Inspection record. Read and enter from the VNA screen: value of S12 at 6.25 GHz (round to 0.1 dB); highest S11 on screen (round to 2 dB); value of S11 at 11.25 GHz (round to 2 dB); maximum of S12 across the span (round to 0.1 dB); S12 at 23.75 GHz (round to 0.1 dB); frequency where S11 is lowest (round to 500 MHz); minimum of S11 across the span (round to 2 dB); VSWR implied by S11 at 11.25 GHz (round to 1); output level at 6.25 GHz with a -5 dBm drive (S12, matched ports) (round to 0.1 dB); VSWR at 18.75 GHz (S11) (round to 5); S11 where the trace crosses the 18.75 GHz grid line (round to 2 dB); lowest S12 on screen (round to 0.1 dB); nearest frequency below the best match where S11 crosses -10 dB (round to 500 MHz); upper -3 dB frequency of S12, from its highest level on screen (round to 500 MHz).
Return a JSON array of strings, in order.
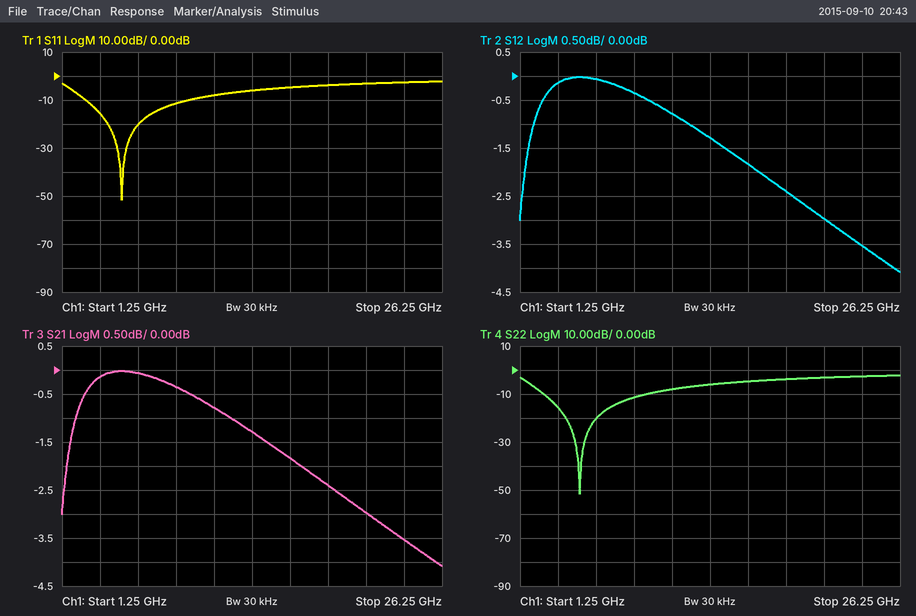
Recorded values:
["-0.1 dB", "-2 dB", "-8 dB", "0.0 dB", "-3.5 dB", "5.0 GHz", "-52 dB", "2", "-5.1 dBm", "5", "-4 dB", "-4.1 dB", "3.0 GHz", "21.5 GHz"]
